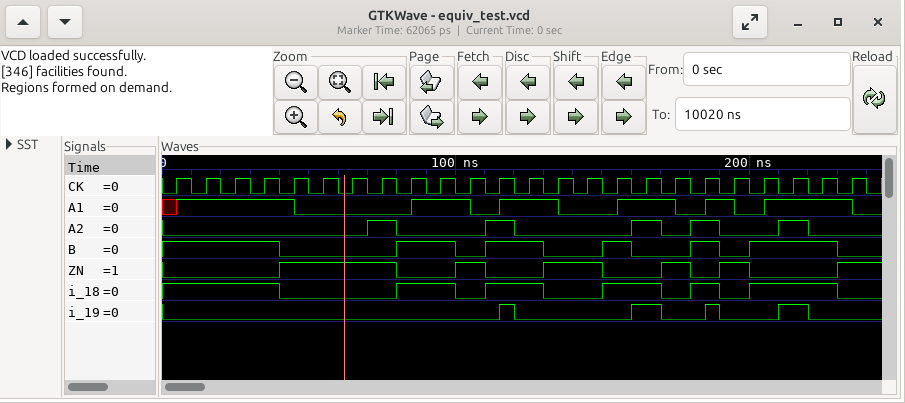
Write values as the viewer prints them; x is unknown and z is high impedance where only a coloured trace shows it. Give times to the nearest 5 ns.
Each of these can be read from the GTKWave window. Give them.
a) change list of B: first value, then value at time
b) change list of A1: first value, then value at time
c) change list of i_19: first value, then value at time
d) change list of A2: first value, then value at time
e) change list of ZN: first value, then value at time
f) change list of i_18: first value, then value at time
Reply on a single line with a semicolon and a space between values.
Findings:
1, 0 at 40 ns, 1 at 80 ns, 0 at 100 ns, 1 at 110 ns, 0 at 130 ns, 1 at 150 ns, 0 at 160 ns, 1 at 180 ns, 0 at 190 ns, 1 at 200 ns, 0 at 230 ns; x, 1 at 5 ns, 0 at 45 ns, 1 at 85 ns, 0 at 105 ns, 1 at 115 ns, 0 at 135 ns, 1 at 155 ns, 0 at 175 ns, 1 at 185 ns, 0 at 195 ns, 1 at 205 ns, 0 at 235 ns; 0, 1 at 115 ns, 0 at 120 ns, 1 at 160 ns, 0 at 170 ns, 1 at 185 ns, 0 at 190 ns, 1 at 210 ns, 0 at 220 ns; 0, 1 at 70 ns, 0 at 80 ns, 1 at 110 ns, 0 at 120 ns, 1 at 160 ns, 0 at 170 ns, 1 at 180 ns, 0 at 190 ns, 1 at 210 ns, 0 at 220 ns; 0, 1 at 40 ns, 0 at 80 ns, 1 at 100 ns, 0 at 110 ns, 1 at 130 ns, 0 at 150 ns, 1 at 170 ns, 0 at 180 ns, 1 at 190 ns, 0 at 200 ns, 1 at 230 ns; 1, 0 at 40 ns, 1 at 80 ns, 0 at 100 ns, 1 at 110 ns, 0 at 130 ns, 1 at 150 ns, 0 at 170 ns, 1 at 180 ns, 0 at 190 ns, 1 at 200 ns, 0 at 230 ns
